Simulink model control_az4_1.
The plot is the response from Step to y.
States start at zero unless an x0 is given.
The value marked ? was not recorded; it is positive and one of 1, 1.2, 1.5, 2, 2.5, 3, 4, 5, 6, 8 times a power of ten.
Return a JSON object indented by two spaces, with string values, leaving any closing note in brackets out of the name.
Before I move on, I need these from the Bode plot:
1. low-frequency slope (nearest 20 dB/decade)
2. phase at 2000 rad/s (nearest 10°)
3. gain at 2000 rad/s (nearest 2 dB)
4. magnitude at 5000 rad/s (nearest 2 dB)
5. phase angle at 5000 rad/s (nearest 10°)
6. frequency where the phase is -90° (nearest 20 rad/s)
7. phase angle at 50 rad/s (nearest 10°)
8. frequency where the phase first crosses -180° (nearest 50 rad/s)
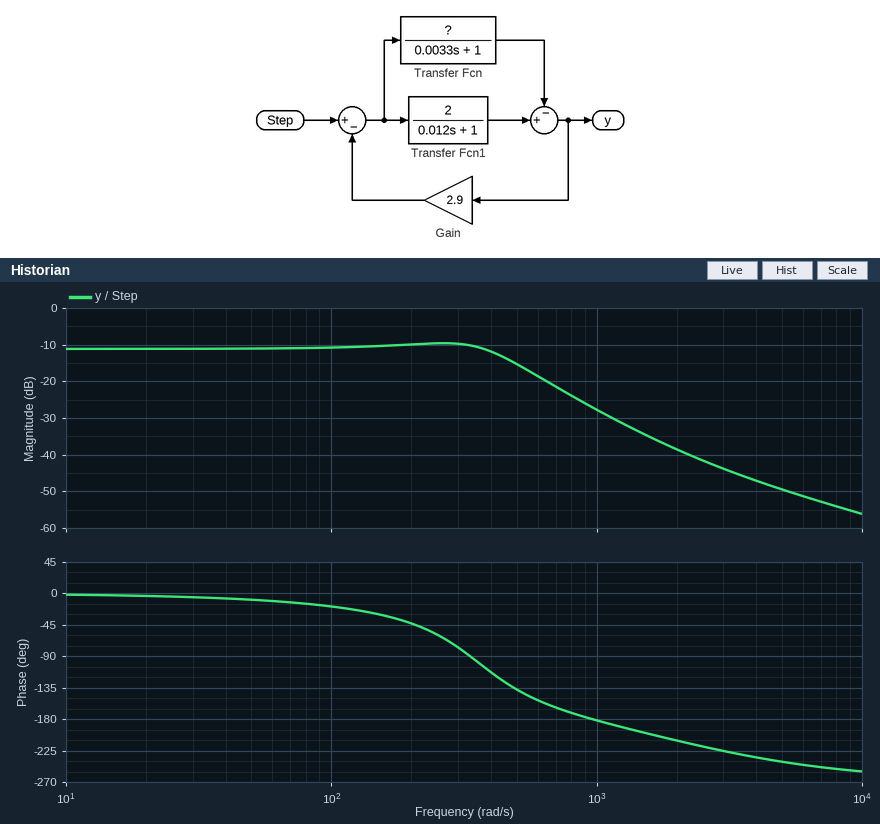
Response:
{
  "low-frequency slope": "0 dB/decade",
  "phase at 2000 rad/s": "-210°",
  "gain at 2000 rad/s": "-38 dB",
  "magnitude at 5000 rad/s": "-50 dB",
  "phase angle at 5000 rad/s": "-240°",
  "frequency where the phase is -90°": "340 rad/s",
  "phase angle at 50 rad/s": "-10°",
  "frequency where the phase first crosses -180°": "950 rad/s"
}
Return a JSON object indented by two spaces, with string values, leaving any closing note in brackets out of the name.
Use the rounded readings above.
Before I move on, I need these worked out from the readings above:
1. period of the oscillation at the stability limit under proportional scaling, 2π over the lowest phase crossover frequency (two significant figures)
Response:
{
  "period of the oscillation at the stability limit under proportional scaling, 2π over the lowest phase crossover frequency": "0.0066 s"
}
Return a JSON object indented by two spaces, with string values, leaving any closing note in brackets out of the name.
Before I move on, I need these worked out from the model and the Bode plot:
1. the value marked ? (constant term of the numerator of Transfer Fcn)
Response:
{
  "the value marked ?": "0.6"
}
